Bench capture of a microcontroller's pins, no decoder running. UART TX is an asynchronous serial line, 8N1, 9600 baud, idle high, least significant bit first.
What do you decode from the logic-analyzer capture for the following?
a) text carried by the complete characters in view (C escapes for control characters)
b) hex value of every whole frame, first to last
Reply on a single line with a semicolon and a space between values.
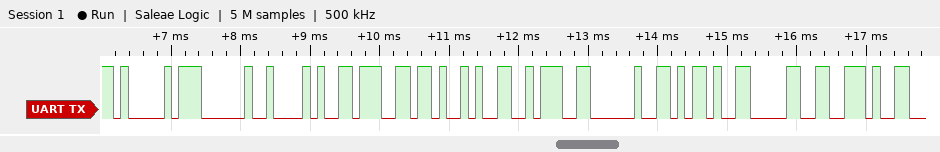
"A (g): -0."; 0x41 0x20 0x28 0x67 0x29 0x3A 0x20 0x2D 0x30 0x2E
